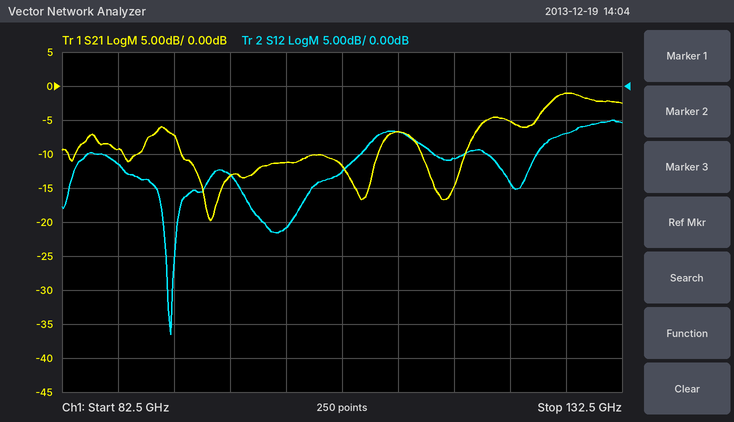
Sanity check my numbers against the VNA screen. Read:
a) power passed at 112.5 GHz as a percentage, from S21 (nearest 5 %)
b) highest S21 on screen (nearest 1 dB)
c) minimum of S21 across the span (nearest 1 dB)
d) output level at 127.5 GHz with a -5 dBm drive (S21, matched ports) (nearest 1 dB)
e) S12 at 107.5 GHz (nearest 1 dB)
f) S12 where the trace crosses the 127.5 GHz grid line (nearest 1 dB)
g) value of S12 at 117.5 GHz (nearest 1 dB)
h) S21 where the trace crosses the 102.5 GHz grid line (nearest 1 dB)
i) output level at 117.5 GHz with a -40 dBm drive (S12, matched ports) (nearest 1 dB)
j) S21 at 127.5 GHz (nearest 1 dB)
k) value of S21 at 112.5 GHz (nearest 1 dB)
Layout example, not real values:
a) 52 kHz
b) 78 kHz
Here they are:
a) 20 %
b) -1 dB
c) -20 dB
d) -6 dBm
e) -13 dB
f) -7 dB
g) -11 dB
h) -11 dB
i) -51 dBm
j) -1 dB
k) -7 dB
